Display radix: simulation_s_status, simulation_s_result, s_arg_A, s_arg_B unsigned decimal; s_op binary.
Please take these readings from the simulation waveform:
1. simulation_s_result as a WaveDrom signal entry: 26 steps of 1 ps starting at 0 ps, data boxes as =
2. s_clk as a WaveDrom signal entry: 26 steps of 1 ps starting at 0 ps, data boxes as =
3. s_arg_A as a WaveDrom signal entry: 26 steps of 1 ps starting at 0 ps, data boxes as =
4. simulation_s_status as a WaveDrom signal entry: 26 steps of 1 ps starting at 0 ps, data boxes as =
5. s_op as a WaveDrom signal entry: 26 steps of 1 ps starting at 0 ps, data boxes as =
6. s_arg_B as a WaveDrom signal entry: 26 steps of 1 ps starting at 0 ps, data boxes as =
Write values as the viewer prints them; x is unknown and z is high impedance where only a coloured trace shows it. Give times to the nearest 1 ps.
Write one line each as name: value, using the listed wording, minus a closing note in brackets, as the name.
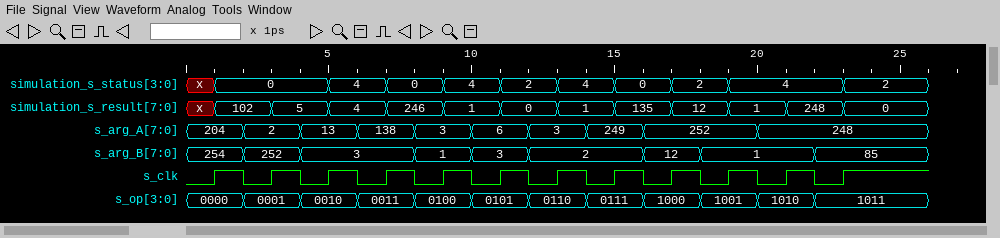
simulation_s_result as a WaveDrom signal entry: 26 steps of 1 ps starting at 0 ps, data boxes as =: {name: 'simulation_s_result', wave: 'x=.=.=.=.=.=.=.=.=.=.=.=..', data: '102 5 4 246 1 0 1 135 12 1 248 0'}
s_clk as a WaveDrom signal entry: 26 steps of 1 ps starting at 0 ps, data boxes as =: {name: 's_clk', wave: '010101010101010101010101..'}
s_arg_A as a WaveDrom signal entry: 26 steps of 1 ps starting at 0 ps, data boxes as =: {name: 's_arg_A', wave: '=.=.=.=.=.=.=.=.=...=.....', data: '204 2 13 138 3 6 3 249 252 248'}
simulation_s_status as a WaveDrom signal entry: 26 steps of 1 ps starting at 0 ps, data boxes as =: {name: 'simulation_s_status', wave: 'x=...=.=.=.=.=.=.=.=...=..', data: '0 4 0 4 2 4 0 2 4 2'}
s_op as a WaveDrom signal entry: 26 steps of 1 ps starting at 0 ps, data boxes as =: {name: 's_op', wave: '=.=.=.=.=.=.=.=.=.=.=.=...', data: '0000 0001 0010 0011 0100 0101 0110 0111 1000 1001 1010 1011'}
s_arg_B as a WaveDrom signal entry: 26 steps of 1 ps starting at 0 ps, data boxes as =: {name: 's_arg_B', wave: '=.=.=...=.=.=...=.=...=...', data: '254 252 3 1 3 2 12 1 85'}
